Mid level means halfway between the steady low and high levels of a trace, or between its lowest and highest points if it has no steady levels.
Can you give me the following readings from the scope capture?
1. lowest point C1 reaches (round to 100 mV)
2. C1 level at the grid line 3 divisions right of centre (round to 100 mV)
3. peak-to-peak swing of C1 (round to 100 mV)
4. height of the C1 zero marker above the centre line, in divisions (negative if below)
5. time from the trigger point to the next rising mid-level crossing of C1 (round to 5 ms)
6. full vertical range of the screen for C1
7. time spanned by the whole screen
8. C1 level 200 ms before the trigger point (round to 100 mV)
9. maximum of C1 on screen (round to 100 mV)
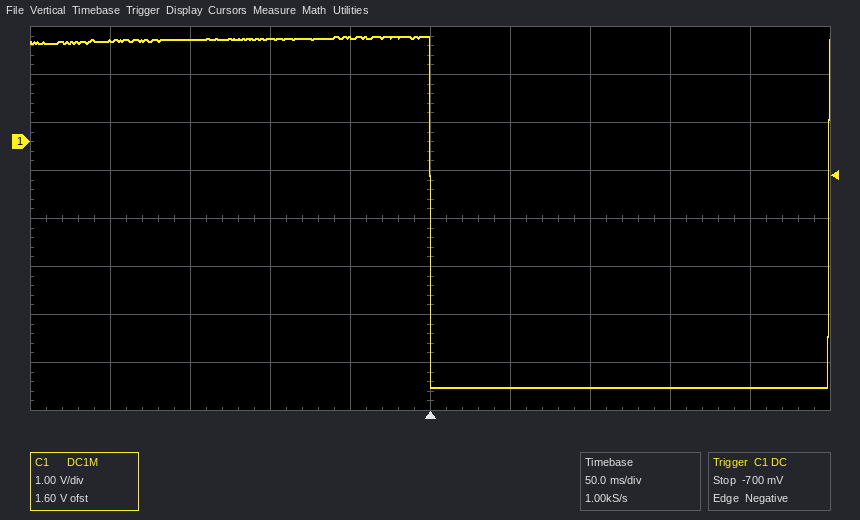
-5.1 V
-5.1 V
7.3 V
+1.6 div
250 ms
8 V
500 ms
2.1 V
2.2 V
